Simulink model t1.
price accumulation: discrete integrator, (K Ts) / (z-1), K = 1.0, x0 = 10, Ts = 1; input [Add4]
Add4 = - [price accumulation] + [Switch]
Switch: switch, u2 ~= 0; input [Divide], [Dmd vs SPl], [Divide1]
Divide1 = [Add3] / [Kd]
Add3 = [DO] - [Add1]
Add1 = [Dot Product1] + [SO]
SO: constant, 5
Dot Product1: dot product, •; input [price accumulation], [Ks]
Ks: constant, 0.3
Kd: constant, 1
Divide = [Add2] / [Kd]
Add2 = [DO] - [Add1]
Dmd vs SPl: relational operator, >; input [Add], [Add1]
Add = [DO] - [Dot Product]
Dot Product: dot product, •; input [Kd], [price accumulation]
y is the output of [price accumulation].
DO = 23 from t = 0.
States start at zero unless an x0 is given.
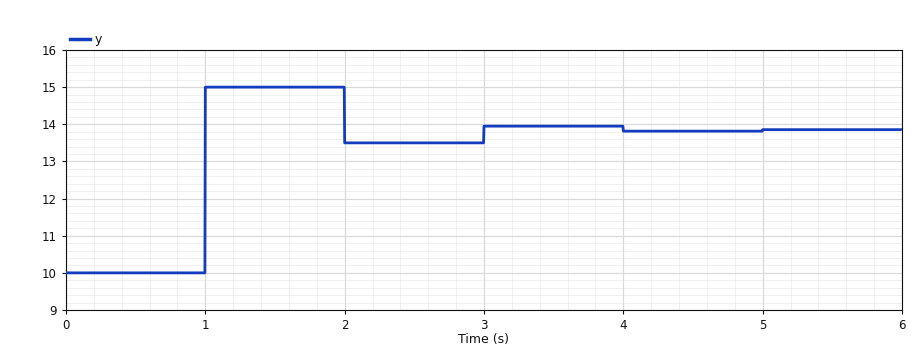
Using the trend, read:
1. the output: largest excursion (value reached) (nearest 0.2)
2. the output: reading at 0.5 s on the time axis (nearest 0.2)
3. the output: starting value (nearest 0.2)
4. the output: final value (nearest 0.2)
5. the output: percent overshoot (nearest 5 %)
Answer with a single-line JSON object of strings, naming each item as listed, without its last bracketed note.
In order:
{"the output: largest excursion (value reached)": "15.0", "the output: reading at 0.5 s on the time axis": "10.0", "the output: starting value": "10.0", "the output: final value": "13.8", "the output: percent overshoot": "30 %"}
